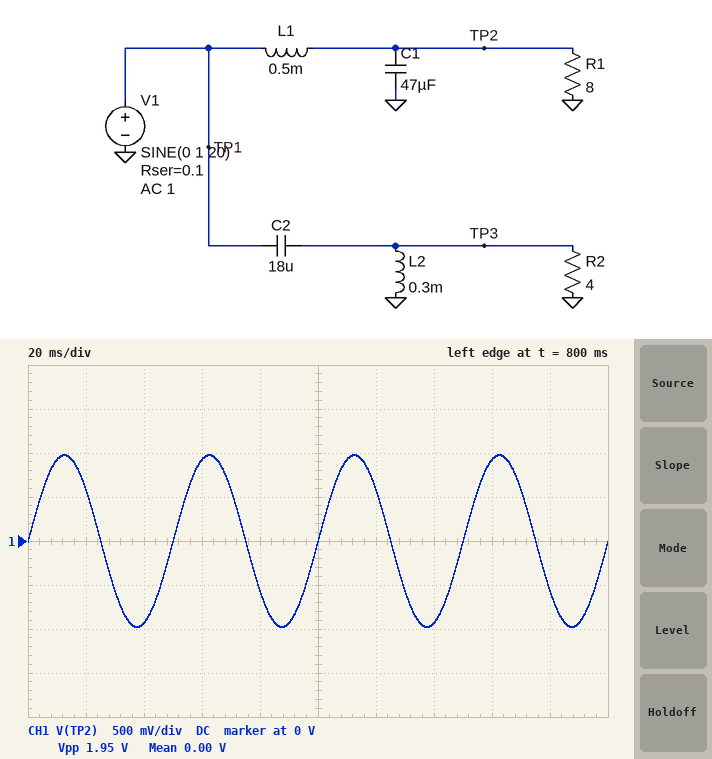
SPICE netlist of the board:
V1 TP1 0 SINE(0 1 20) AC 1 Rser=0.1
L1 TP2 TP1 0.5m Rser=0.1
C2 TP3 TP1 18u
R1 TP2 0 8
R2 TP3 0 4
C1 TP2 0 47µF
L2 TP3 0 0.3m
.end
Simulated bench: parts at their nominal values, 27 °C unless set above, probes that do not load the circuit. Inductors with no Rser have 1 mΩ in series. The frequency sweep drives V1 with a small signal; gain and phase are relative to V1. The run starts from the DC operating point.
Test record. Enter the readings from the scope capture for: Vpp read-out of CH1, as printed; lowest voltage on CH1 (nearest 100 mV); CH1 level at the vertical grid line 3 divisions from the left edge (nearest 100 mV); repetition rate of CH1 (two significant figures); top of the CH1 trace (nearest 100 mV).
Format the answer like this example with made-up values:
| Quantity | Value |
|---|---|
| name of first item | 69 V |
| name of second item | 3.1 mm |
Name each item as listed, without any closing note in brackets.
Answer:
| Quantity | Value |
|---|---|
| Vpp read-out of CH1, as printed | 1.95 V |
| lowest voltage on CH1 | -1.0 V |
| CH1 level at the vertical grid line 3 divisions from the left edge | 900 mV |
| repetition rate of CH1 | 20 Hz |
| top of the CH1 trace | 1.0 V |
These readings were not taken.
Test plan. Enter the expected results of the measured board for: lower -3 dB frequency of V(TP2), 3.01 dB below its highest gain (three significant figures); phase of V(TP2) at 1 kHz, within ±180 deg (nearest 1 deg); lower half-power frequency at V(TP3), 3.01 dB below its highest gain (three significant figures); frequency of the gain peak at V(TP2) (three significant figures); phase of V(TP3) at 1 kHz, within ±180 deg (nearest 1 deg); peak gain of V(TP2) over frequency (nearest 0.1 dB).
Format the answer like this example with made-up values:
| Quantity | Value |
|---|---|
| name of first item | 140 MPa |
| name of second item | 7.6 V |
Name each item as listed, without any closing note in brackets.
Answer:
| Quantity | Value |
|---|---|
| lower -3 dB frequency of V(TP2), 3.01 dB below its highest gain | 698 Hz |
| phase of V(TP2) at 1 kHz, within ±180 deg | -79 deg |
| lower half-power frequency at V(TP3), 3.01 dB below its highest gain | 1.84 kHz |
| frequency of the gain peak at V(TP2) | 993 Hz |
| phase of V(TP3) at 1 kHz, within ±180 deg | 149 deg |
| peak gain of V(TP2) over frequency | 6.7 dB |
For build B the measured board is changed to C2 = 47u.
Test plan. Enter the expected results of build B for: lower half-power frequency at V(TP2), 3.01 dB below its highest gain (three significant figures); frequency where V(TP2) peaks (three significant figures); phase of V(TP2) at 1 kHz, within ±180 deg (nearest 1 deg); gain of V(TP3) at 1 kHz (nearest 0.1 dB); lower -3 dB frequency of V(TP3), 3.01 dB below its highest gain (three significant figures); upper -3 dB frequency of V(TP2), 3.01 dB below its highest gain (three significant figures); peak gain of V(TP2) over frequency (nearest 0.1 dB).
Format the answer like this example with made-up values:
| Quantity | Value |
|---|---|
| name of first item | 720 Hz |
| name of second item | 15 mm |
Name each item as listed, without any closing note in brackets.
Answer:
| Quantity | Value |
|---|---|
| lower half-power frequency at V(TP2), 3.01 dB below its highest gain | 689 Hz |
| frequency where V(TP2) peaks | 988 Hz |
| phase of V(TP2) at 1 kHz, within ±180 deg | -80 deg |
| gain of V(TP3) at 1 kHz | -2.1 dB |
| lower -3 dB frequency of V(TP3), 3.01 dB below its highest gain | 1.14 kHz |
| upper -3 dB frequency of V(TP2), 3.01 dB below its highest gain | 1.21 kHz |
| peak gain of V(TP2) over frequency | 6.6 dB |
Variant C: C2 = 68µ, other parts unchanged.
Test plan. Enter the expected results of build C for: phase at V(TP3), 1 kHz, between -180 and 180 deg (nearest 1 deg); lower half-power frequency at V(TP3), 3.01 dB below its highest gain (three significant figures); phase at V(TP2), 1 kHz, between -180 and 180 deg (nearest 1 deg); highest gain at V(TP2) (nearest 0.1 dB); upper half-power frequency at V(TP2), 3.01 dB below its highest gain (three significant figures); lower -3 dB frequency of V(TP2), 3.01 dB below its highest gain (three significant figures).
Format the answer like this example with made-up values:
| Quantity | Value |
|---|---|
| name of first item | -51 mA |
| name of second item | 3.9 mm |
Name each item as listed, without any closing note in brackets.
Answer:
| Quantity | Value |
|---|---|
| phase at V(TP3), 1 kHz, between -180 and 180 deg | 110 deg |
| lower half-power frequency at V(TP3), 3.01 dB below its highest gain | 948 Hz |
| phase at V(TP2), 1 kHz, between -180 and 180 deg | -81 deg |
| highest gain at V(TP2) | 6.2 dB |
| upper half-power frequency at V(TP2), 3.01 dB below its highest gain | 1.20 kHz |
| lower -3 dB frequency of V(TP2), 3.01 dB below its highest gain | 665 Hz |
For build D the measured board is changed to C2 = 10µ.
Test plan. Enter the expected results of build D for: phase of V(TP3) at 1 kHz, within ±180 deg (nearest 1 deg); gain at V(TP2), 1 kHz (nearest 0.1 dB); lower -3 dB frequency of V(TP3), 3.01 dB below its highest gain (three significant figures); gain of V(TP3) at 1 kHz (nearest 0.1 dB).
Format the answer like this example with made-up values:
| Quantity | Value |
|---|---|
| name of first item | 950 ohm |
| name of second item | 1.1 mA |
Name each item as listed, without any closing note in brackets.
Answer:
| Quantity | Value |
|---|---|
| phase of V(TP3) at 1 kHz, within ±180 deg | 152 deg |
| gain at V(TP2), 1 kHz | 6.7 dB |
| lower -3 dB frequency of V(TP3), 3.01 dB below its highest gain | 2.79 kHz |
| gain of V(TP3) at 1 kHz | -19.1 dB |
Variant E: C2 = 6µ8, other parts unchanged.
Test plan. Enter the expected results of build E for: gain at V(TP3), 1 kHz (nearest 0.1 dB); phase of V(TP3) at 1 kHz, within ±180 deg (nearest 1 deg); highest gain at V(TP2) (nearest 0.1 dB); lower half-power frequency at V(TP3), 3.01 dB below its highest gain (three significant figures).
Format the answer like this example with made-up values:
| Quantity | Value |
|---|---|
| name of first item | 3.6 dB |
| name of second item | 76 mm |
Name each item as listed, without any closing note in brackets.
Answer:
| Quantity | Value |
|---|---|
| gain at V(TP3), 1 kHz | -22.8 dB |
| phase of V(TP3) at 1 kHz, within ±180 deg | 153 deg |
| highest gain at V(TP2) | 6.7 dB |
| lower half-power frequency at V(TP3), 3.01 dB below its highest gain | 4.17 kHz |
